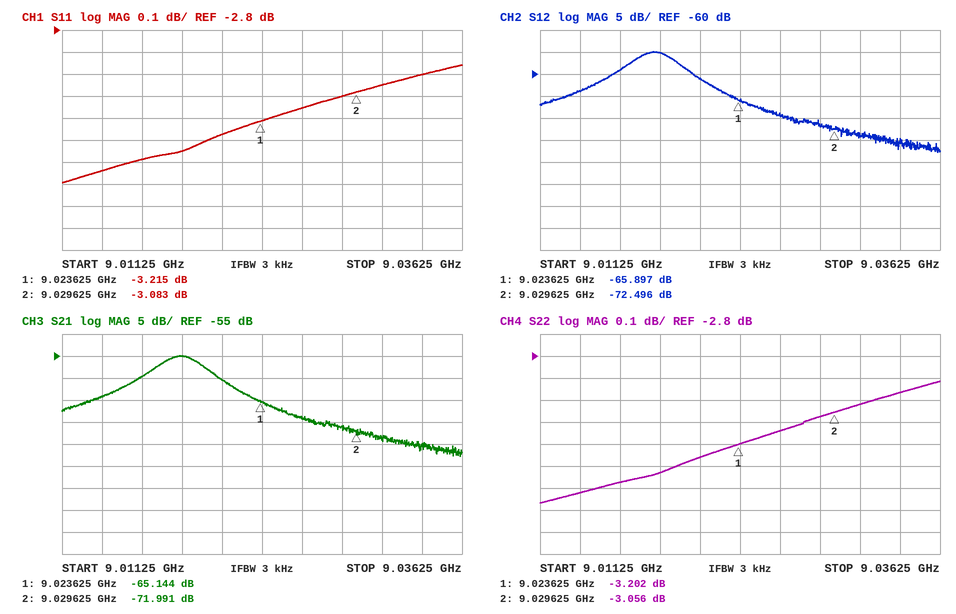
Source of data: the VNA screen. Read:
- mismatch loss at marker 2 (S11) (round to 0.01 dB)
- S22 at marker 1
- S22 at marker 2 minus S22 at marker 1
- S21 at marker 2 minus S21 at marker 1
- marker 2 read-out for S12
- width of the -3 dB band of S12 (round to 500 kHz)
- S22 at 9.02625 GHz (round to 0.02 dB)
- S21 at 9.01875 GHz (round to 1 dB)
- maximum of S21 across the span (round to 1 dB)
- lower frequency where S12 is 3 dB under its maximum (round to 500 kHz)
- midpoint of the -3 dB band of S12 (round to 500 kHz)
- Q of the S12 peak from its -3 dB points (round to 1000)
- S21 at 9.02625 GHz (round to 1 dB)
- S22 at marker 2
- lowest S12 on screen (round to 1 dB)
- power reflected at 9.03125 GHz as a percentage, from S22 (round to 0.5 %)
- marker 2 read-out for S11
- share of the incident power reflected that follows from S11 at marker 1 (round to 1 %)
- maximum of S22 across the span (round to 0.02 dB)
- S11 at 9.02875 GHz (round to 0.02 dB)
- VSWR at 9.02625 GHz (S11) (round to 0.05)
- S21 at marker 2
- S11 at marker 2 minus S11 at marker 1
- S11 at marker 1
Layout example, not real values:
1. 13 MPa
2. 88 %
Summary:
1. 2.94 dB
2. -3.202 dB
3. 0.146 dB
4. -6.847 dB
5. -72.496 dB
6. 3.5 MHz
7. -3.14 dB
8. -55 dB
9. -55 dB
10. 9.0165 GHz
11. 9.0185 GHz
12. 3000
13. -69 dB
14. -3.056 dB
15. -78 dB
16. 50.0 %
17. -3.083 dB
18. 48 %
19. -2.92 dB
20. -3.10 dB
21. 5.55
22. -71.991 dB
23. 0.132 dB
24. -3.215 dB
